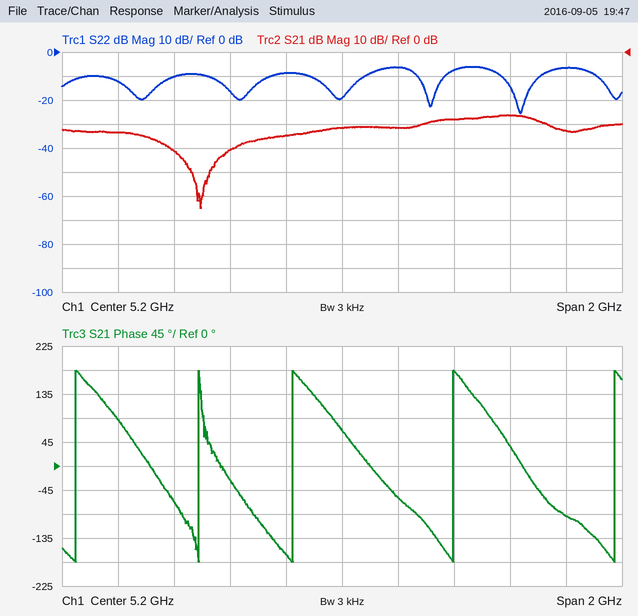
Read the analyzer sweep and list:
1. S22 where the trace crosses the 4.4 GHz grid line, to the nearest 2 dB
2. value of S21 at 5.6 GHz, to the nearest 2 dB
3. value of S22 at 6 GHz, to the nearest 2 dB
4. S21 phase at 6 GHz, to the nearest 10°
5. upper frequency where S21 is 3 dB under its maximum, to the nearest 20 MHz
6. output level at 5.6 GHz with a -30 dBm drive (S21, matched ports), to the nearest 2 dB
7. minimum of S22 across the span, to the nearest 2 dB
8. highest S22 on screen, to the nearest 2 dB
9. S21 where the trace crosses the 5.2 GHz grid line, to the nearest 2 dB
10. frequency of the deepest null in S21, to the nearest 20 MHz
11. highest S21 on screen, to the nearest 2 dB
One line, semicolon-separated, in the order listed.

-12 dB; -28 dB; -6 dB; -90°; 5.92 GHz; -58 dBm; -26 dB; -6 dB; -32 dB; 4.70 GHz; -26 dB
